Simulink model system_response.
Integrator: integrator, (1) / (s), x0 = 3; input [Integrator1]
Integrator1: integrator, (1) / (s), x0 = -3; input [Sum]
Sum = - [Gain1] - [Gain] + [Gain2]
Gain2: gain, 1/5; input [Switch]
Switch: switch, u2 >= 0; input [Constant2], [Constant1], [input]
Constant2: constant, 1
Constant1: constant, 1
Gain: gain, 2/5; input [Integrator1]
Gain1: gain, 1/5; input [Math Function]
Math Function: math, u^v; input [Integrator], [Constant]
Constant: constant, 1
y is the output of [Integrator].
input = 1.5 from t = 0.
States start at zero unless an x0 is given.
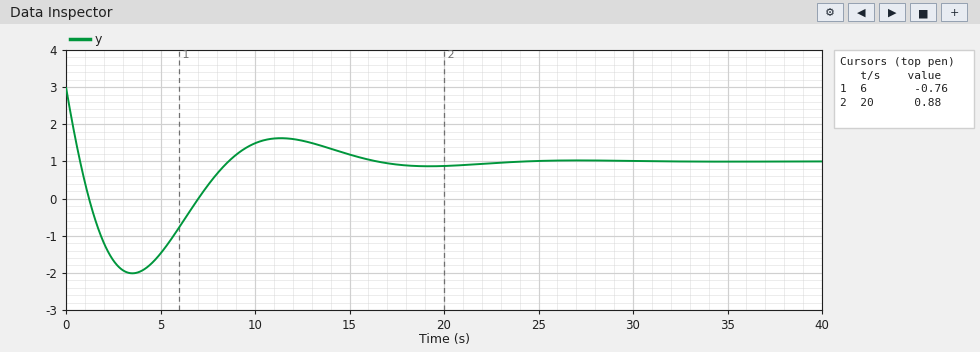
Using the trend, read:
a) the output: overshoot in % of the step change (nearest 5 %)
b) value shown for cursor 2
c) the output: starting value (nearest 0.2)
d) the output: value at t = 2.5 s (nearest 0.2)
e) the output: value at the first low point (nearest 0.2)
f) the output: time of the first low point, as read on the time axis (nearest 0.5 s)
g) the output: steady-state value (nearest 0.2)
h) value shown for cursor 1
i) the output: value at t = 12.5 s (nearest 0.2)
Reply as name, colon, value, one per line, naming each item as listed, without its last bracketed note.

the output: overshoot in % of the step change: 150 %
value shown for cursor 2: 0.88
the output: starting value: 3.0
the output: value at t = 2.5 s: -1.6
the output: value at the first low point: -2.0
the output: time of the first low point, as read on the time axis: 3.5 s
the output: steady-state value: 1.0
value shown for cursor 1: -0.76
the output: value at t = 12.5 s: 1.6
